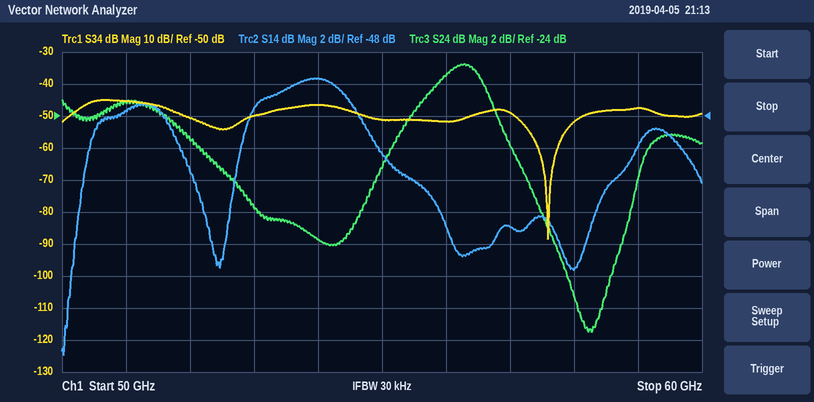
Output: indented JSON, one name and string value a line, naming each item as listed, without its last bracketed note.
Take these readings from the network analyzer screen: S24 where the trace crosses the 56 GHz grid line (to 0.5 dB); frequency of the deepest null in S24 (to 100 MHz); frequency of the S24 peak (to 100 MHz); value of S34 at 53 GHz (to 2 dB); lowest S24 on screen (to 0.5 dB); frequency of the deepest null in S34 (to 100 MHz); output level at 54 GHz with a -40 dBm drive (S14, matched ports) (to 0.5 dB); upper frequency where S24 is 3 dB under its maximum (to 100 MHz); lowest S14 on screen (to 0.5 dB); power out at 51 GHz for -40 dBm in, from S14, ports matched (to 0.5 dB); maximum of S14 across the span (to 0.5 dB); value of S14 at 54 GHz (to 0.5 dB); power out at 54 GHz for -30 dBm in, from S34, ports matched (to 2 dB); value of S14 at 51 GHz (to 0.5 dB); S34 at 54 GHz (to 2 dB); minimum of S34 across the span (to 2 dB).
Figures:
{
  "S24 where the trace crosses the 56 GHz grid line": "-21.5 dB",
  "frequency of the deepest null in S24": "58.2 GHz",
  "frequency of the S24 peak": "56.3 GHz",
  "value of S34 at 53 GHz": "-50 dB",
  "lowest S24 on screen": "-37.5 dB",
  "frequency of the deepest null in S34": "57.6 GHz",
  "output level at 54 GHz with a -40 dBm drive (S14, matched ports)": "-85.5 dBm",
  "upper frequency where S24 is 3 dB under its maximum": "56.8 GHz",
  "lowest S14 on screen": "-63.0 dB",
  "power out at 51 GHz for -40 dBm in, from S14, ports matched": "-87.5 dBm",
  "maximum of S14 across the span": "-45.5 dB",
  "value of S14 at 54 GHz": "-45.5 dB",
  "power out at 54 GHz for -30 dBm in, from S34, ports matched": "-76 dBm",
  "value of S14 at 51 GHz": "-47.5 dB",
  "S34 at 54 GHz": "-46 dB",
  "minimum of S34 across the span": "-88 dB"
}
